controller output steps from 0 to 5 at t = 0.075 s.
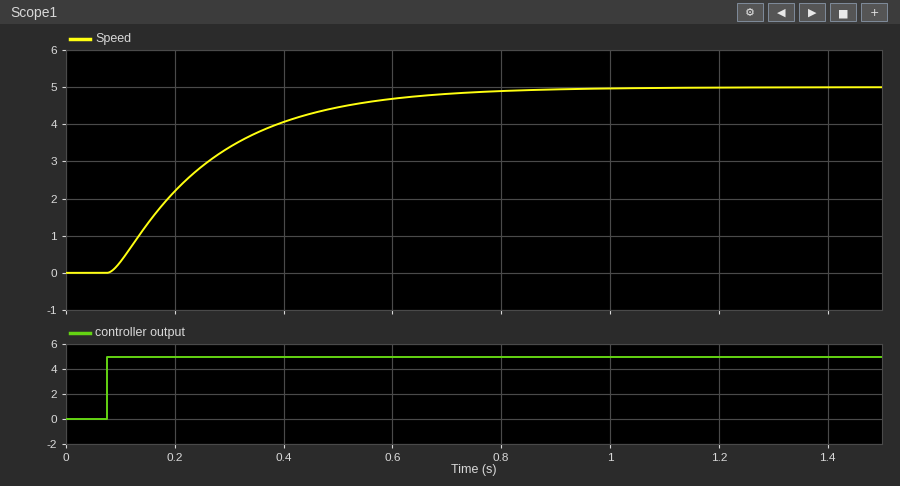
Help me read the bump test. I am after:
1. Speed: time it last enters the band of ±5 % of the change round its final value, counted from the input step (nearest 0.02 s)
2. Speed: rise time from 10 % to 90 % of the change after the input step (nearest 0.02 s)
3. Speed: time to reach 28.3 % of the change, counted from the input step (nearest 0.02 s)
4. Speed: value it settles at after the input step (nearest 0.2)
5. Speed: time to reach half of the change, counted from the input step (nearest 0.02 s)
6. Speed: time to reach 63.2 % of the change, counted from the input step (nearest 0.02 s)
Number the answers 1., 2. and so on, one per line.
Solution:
1. 0.56 s
2. 0.40 s
3. 0.08 s
4. 5.0
5. 0.14 s
6. 0.20 s
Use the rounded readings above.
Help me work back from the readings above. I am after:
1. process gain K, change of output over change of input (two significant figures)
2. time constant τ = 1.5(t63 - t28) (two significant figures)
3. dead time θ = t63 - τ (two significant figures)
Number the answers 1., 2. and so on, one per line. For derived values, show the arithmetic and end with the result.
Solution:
1. (5 - 0) / 5 = 1.0
2. 1.5 × (0.2 - 0.08) = 0.18 s
3. 0.2 - 0.18 = 0.020 s
